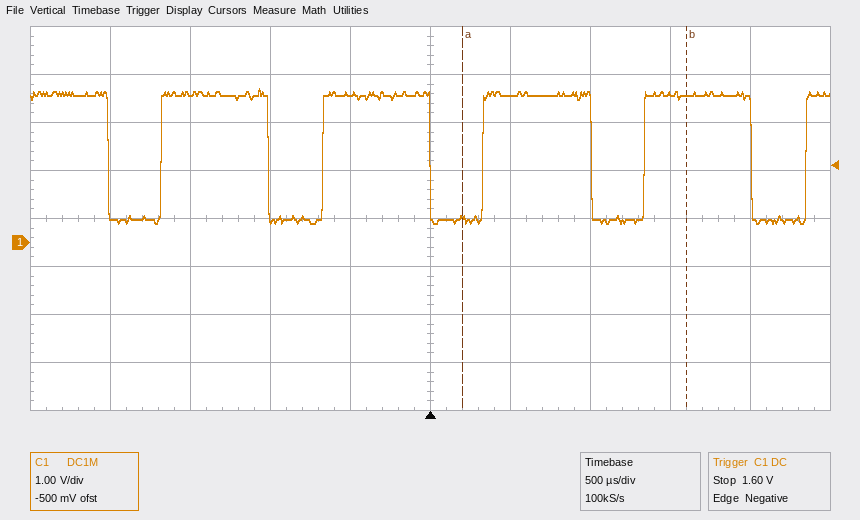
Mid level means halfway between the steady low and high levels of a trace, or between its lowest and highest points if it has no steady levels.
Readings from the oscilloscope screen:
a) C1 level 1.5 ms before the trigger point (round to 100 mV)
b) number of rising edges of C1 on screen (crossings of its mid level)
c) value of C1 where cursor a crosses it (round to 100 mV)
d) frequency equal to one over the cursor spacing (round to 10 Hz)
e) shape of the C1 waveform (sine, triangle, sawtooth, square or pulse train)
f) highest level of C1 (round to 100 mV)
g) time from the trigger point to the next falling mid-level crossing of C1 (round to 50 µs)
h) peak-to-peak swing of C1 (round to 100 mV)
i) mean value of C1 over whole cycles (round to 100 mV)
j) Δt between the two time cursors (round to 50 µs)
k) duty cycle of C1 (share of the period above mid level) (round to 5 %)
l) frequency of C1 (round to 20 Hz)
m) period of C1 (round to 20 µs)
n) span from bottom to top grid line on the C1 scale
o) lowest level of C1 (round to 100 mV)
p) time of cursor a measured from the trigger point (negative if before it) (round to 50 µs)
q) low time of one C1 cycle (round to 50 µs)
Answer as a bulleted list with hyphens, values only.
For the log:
- 3.1 V
- 5
- 500 mV
- 710 Hz
- pulse train
- 3.2 V
- 1.00 ms
- 2.8 V
- 2.2 V
- 1.40 ms
- 65 %
- 1.00 kHz
- 1.00 ms
- 8 V
- 400 mV
- +200 µs
- 350 µs
